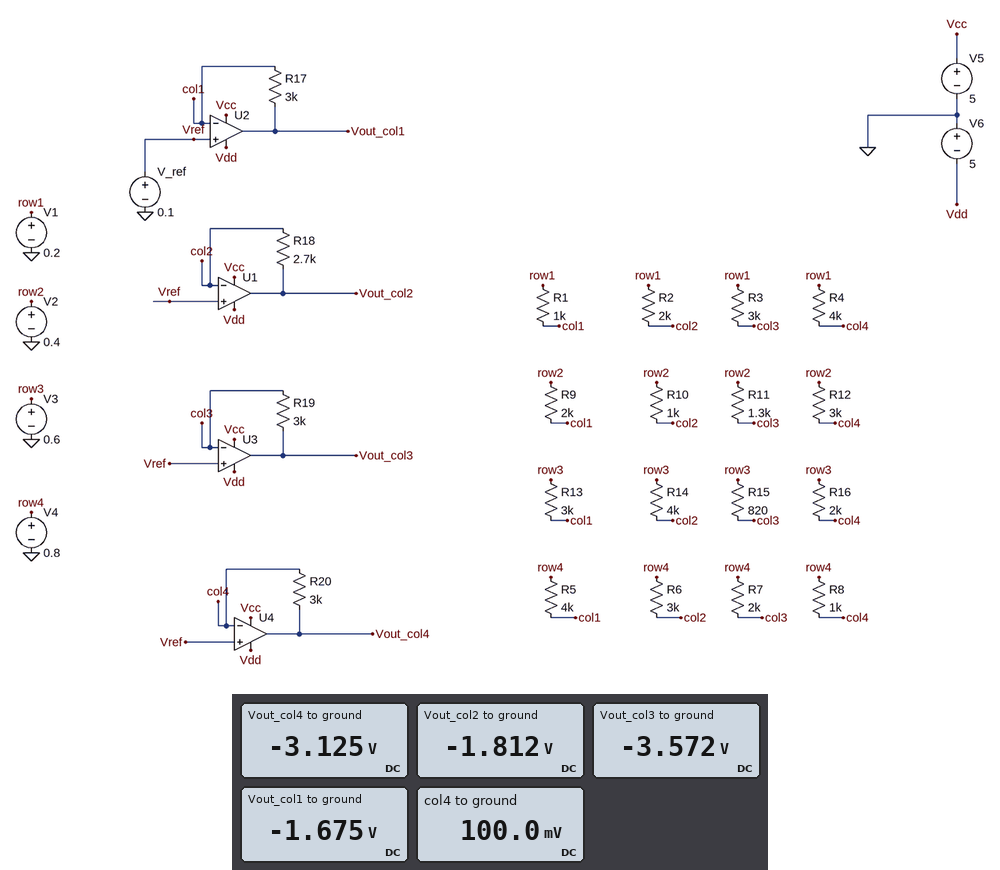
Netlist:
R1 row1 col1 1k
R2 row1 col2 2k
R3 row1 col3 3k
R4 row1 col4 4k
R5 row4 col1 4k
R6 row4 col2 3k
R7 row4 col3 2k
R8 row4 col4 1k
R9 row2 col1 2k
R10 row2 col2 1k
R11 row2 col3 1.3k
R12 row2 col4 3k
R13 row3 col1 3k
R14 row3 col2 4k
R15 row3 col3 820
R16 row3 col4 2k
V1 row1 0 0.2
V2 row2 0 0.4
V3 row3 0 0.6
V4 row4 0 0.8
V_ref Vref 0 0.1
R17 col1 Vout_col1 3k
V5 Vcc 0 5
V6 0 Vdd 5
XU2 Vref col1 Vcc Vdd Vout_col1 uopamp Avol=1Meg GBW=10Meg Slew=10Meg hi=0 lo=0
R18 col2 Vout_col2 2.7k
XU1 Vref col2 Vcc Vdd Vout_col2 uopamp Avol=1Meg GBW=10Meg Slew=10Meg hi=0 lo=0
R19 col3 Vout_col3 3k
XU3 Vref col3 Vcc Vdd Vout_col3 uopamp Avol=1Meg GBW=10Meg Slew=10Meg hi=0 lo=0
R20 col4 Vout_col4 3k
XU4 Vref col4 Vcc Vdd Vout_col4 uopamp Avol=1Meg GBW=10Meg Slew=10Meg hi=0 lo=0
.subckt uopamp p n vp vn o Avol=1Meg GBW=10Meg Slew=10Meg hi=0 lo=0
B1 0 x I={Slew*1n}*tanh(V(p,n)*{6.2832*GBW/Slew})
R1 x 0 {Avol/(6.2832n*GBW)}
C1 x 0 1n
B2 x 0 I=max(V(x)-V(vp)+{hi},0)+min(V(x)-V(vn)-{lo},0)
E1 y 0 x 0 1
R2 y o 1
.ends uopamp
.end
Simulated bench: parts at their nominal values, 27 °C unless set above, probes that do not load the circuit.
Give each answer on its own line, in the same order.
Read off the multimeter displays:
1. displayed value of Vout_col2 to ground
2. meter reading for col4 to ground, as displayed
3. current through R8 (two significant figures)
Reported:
-1.812 V
100.0 mV
700 µA
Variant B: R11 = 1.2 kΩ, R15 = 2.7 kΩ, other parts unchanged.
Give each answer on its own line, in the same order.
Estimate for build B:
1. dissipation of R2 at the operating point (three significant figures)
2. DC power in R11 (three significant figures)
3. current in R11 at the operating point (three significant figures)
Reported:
5.00 µW
75.0 µW
250 µA
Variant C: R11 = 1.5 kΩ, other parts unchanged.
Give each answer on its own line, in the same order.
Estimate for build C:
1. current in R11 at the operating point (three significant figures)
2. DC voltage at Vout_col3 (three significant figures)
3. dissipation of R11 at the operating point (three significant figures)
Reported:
200 µA
-3.48 V
60.0 µW
